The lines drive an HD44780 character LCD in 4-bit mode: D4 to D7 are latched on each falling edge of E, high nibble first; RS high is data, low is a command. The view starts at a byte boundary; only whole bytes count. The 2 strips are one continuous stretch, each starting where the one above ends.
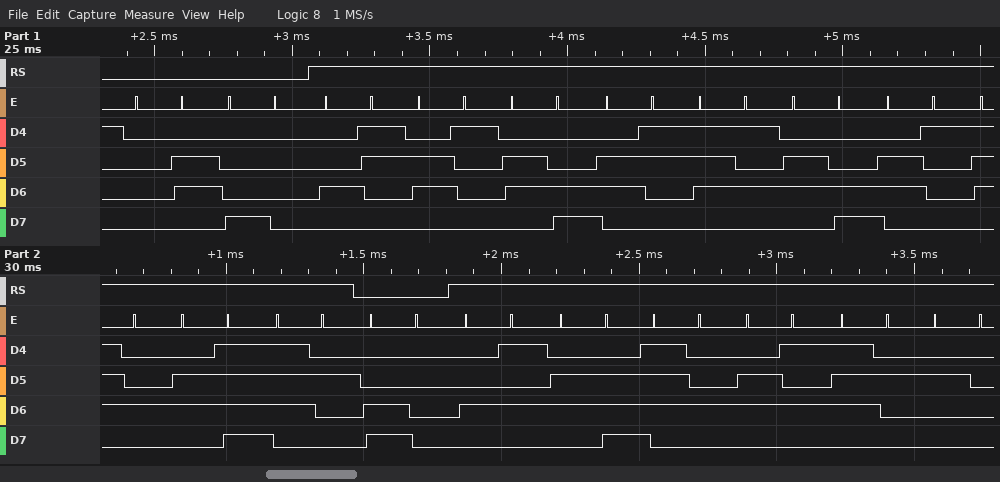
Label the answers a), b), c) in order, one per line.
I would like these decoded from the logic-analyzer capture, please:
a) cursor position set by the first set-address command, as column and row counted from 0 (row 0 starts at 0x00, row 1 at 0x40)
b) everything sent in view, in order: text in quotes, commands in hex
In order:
a) column 0, row 0
b) 0x06 0x80 "Calculator" 0xC0 "Enter "
